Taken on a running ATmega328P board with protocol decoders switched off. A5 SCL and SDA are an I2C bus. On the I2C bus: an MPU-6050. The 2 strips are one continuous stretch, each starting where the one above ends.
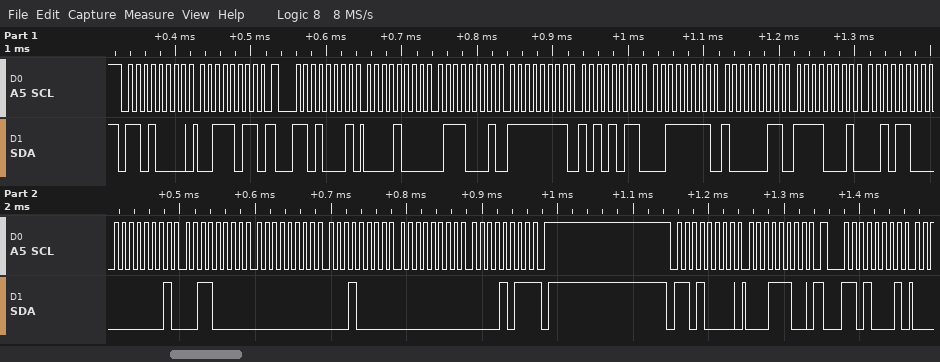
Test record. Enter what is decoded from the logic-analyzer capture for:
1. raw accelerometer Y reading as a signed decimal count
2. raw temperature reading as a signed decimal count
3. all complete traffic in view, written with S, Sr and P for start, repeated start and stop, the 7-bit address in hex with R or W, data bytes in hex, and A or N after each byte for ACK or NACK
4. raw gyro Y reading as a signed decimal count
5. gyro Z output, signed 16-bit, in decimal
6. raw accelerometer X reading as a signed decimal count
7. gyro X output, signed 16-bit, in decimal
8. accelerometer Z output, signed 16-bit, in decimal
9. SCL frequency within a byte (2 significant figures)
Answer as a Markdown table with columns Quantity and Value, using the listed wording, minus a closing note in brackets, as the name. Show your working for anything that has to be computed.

| Quantity | Value |
|---|---|
| raw accelerometer Y reading as a signed decimal count | 0xFFAB = -85 |
| raw temperature reading as a signed decimal count | 0xF12C = -3796 |
| all complete traffic in view, written with S, Sr and P for start, repeated start and stop, the 7-bit address in hex with R or W, data bytes in hex, and A or N after each byte for ACK or NACK | S 68W A 3B A Sr 68R A 08 A 71 A FF A AB A 3F A 83 A F1 A 2C A 01 A 30 A 00 A 10 A 00 A 0B N P S 68W A 1C A Sr 68R A |
| raw gyro Y reading as a signed decimal count | 0x0010 = 16 |
| gyro Z output, signed 16-bit, in decimal | 0x000B = 11 |
| raw accelerometer X reading as a signed decimal count | 0x0871 = 2161 |
| gyro X output, signed 16-bit, in decimal | 0x0130 = 304 |
| accelerometer Z output, signed 16-bit, in decimal | 0x3F83 = 16259 |
| SCL frequency within a byte | 100 kHz |
